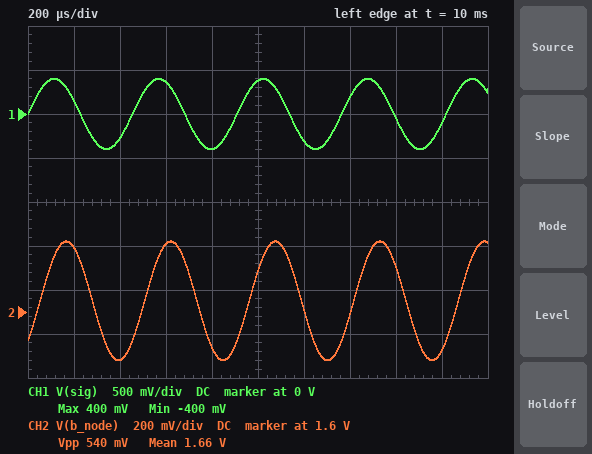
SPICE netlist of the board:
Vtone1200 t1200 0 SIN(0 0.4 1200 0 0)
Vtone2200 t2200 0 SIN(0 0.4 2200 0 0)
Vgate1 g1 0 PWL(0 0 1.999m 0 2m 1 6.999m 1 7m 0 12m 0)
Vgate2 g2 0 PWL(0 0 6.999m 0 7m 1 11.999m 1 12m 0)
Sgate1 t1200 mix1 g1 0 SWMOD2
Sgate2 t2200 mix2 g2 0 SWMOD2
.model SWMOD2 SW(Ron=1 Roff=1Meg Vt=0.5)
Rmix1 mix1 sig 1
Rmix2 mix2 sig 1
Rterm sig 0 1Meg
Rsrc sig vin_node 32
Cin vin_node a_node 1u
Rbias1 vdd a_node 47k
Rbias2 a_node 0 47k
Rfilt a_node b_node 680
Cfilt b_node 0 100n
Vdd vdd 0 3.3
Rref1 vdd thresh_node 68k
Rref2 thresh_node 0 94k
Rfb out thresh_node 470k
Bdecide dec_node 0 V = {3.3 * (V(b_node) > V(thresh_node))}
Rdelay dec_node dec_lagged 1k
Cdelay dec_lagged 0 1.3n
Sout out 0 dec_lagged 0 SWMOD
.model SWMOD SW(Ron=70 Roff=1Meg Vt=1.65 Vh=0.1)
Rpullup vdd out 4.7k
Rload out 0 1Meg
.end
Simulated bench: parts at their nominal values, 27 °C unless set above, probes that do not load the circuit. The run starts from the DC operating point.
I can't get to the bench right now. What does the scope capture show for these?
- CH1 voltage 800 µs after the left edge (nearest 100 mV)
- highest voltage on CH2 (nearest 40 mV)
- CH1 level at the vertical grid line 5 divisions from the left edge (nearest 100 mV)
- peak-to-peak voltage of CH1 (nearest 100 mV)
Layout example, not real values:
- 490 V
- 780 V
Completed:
- -400 mV
- 1.92 V
- 400 mV
- 800 mV
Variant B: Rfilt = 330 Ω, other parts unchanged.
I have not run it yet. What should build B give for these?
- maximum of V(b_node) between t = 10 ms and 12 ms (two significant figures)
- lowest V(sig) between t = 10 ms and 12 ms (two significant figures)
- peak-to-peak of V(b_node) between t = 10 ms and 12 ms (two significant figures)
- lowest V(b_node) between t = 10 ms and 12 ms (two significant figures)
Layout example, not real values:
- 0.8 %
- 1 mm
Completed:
- 2.0 V
- -400 mV
- 660 mV
- 1.3 V
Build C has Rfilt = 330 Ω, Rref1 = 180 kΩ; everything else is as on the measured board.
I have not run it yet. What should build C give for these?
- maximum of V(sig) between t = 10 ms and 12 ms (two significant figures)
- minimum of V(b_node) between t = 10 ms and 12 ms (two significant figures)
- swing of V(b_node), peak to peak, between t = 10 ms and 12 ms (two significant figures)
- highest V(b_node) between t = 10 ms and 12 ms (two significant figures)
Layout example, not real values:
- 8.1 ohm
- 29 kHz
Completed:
- 400 mV
- 1.3 V
- 660 mV
- 2.0 V
